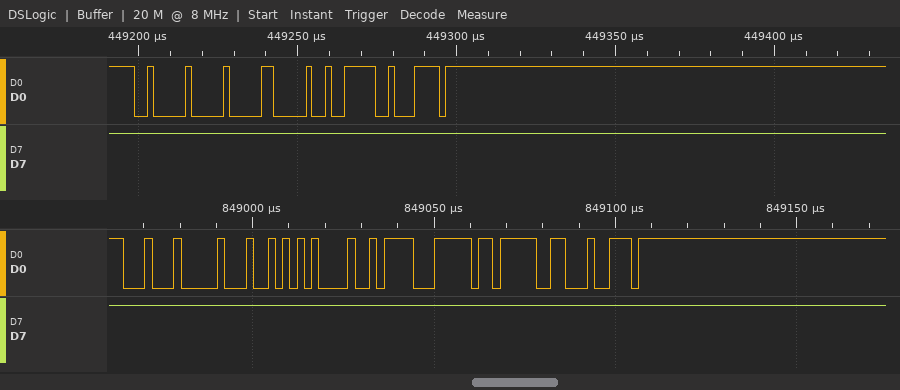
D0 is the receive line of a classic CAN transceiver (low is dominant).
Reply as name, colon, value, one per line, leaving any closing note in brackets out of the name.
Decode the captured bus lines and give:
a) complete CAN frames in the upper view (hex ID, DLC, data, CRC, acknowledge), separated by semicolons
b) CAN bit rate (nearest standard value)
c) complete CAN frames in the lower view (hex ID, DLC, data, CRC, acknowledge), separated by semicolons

complete CAN frames in the upper view (hex ID, DLC, data, CRC, acknowledge), separated by semicolons: ID 200, DLC 1, data 01, CRC 1F47, ACK
CAN bit rate: 500 kbit/s
complete CAN frames in the lower view (hex ID, DLC, data, CRC, acknowledge), separated by semicolons: ID 110, DLC 4, data AA 12 F1 FD, CRC 7B13, ACK
